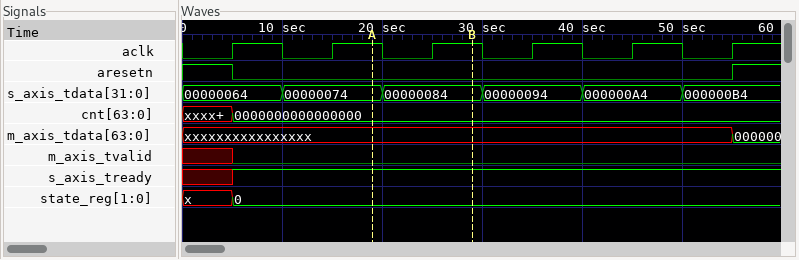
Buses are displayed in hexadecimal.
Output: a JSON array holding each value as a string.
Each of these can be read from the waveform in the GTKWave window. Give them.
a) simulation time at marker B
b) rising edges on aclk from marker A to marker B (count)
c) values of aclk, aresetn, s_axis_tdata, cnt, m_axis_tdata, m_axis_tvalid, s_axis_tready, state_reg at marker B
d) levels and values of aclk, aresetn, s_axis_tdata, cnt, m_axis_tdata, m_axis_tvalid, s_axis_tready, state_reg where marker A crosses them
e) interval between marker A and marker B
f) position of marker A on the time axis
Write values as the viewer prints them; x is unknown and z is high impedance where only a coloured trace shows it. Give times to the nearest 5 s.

["30 s", "1", "aclk=1, aresetn=0, s_axis_tdata=00000084, cnt=0000000000000000, m_axis_tdata=xxxxxxxxxxxxxxxx, m_axis_tvalid=0, s_axis_tready=1, state_reg=0", "aclk=1, aresetn=0, s_axis_tdata=00000074, cnt=0000000000000000, m_axis_tdata=xxxxxxxxxxxxxxxx, m_axis_tvalid=0, s_axis_tready=1, state_reg=0", "10 s", "20 s"]
